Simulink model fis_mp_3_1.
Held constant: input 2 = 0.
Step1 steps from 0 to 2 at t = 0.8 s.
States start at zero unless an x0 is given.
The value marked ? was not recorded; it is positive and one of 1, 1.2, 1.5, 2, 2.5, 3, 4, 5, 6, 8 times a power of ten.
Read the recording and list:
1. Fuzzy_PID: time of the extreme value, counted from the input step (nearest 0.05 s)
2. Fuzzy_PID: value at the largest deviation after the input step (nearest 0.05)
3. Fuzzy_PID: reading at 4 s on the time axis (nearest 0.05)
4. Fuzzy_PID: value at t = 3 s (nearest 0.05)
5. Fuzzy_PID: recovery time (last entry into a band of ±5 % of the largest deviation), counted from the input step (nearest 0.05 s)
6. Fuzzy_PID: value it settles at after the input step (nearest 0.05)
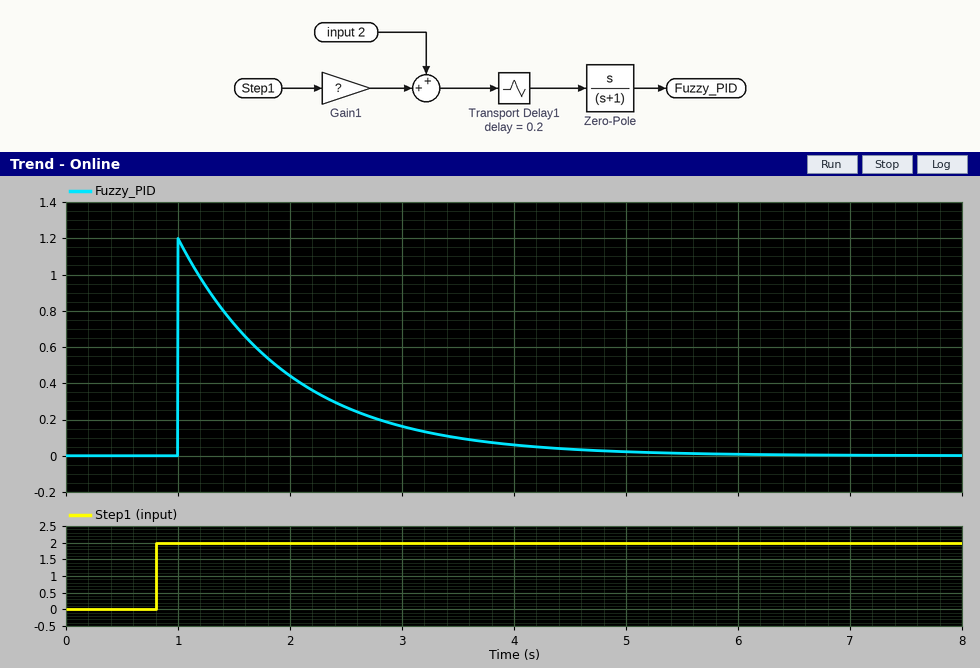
0.20 s
1.20
0.05
0.15
3.20 s
0.00
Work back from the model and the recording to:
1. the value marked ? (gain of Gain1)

0.6
